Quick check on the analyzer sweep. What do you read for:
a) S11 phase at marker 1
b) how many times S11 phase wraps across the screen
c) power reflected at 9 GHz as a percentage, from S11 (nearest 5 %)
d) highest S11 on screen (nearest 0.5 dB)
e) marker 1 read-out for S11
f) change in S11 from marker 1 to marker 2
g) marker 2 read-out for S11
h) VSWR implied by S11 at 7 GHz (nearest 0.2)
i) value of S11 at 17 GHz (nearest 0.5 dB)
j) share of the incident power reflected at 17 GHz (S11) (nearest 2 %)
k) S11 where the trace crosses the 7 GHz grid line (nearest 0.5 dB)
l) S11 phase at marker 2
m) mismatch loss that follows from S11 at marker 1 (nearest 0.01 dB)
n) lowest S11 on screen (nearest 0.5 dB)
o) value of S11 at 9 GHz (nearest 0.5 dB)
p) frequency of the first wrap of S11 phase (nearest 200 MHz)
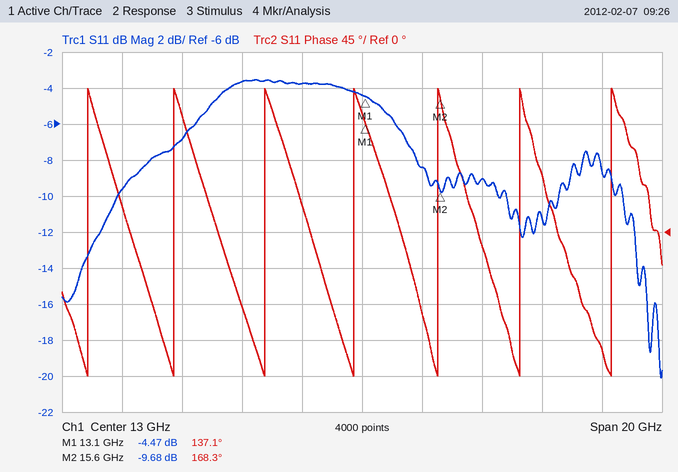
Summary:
137.1°
7
45 %
-3.5 dB
-4.47 dB
-5.21 dB
-9.68 dB
2.6
-9.0 dB
12 %
-7.0 dB
168.3°
1.92 dB
-20.0 dB
-3.5 dB
3.8 GHz
